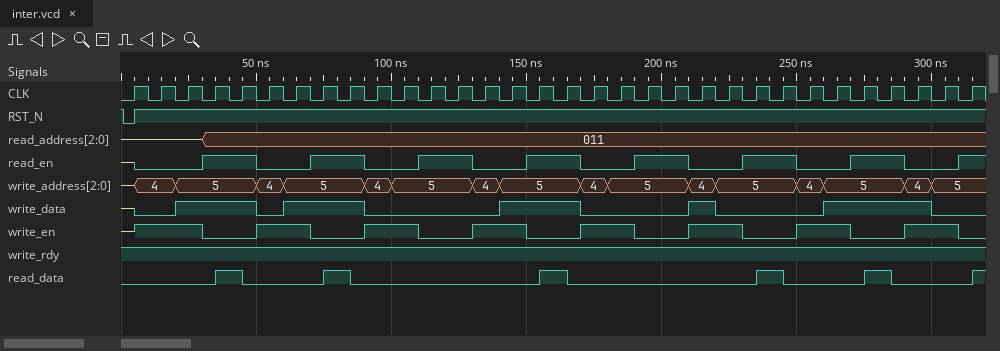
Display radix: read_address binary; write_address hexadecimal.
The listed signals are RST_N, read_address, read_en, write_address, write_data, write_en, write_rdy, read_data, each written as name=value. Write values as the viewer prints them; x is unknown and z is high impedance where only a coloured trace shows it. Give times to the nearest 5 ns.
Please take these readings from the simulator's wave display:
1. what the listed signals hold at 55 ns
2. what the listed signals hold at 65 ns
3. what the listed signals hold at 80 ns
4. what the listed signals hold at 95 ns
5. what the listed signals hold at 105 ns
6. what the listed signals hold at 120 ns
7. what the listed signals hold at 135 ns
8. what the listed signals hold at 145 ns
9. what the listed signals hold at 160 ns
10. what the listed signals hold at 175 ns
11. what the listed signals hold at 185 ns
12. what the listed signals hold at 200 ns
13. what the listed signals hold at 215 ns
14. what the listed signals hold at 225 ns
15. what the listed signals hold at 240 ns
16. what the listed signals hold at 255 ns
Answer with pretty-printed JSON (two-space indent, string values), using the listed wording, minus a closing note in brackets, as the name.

{
  "what the listed signals hold at 55 ns": "RST_N=1, read_address=011, read_en=0, write_address=4, write_data=0, write_en=1, write_rdy=1, read_data=0",
  "what the listed signals hold at 65 ns": "RST_N=1, read_address=011, read_en=0, write_address=5, write_data=1, write_en=1, write_rdy=1, read_data=0",
  "what the listed signals hold at 80 ns": "RST_N=1, read_address=011, read_en=1, write_address=5, write_data=1, write_en=0, write_rdy=1, read_data=1",
  "what the listed signals hold at 95 ns": "RST_N=1, read_address=011, read_en=0, write_address=4, write_data=0, write_en=1, write_rdy=1, read_data=0",
  "what the listed signals hold at 105 ns": "RST_N=1, read_address=011, read_en=0, write_address=5, write_data=0, write_en=1, write_rdy=1, read_data=0",
  "what the listed signals hold at 120 ns": "RST_N=1, read_address=011, read_en=1, write_address=5, write_data=0, write_en=0, write_rdy=1, read_data=0",
  "what the listed signals hold at 135 ns": "RST_N=1, read_address=011, read_en=0, write_address=4, write_data=0, write_en=1, write_rdy=1, read_data=0",
  "what the listed signals hold at 145 ns": "RST_N=1, read_address=011, read_en=0, write_address=5, write_data=1, write_en=1, write_rdy=1, read_data=0",
  "what the listed signals hold at 160 ns": "RST_N=1, read_address=011, read_en=1, write_address=5, write_data=1, write_en=0, write_rdy=1, read_data=1",
  "what the listed signals hold at 175 ns": "RST_N=1, read_address=011, read_en=0, write_address=4, write_data=0, write_en=1, write_rdy=1, read_data=0",
  "what the listed signals hold at 185 ns": "RST_N=1, read_address=011, read_en=0, write_address=5, write_data=0, write_en=1, write_rdy=1, read_data=0",
  "what the listed signals hold at 200 ns": "RST_N=1, read_address=011, read_en=1, write_address=5, write_data=0, write_en=0, write_rdy=1, read_data=0",
  "what the listed signals hold at 215 ns": "RST_N=1, read_address=011, read_en=0, write_address=4, write_data=1, write_en=1, write_rdy=1, read_data=0",
  "what the listed signals hold at 225 ns": "RST_N=1, read_address=011, read_en=0, write_address=5, write_data=0, write_en=1, write_rdy=1, read_data=0",
  "what the listed signals hold at 240 ns": "RST_N=1, read_address=011, read_en=1, write_address=5, write_data=0, write_en=0, write_rdy=1, read_data=1",
  "what the listed signals hold at 255 ns": "RST_N=1, read_address=011, read_en=0, write_address=4, write_data=0, write_en=1, write_rdy=1, read_data=0"
}
